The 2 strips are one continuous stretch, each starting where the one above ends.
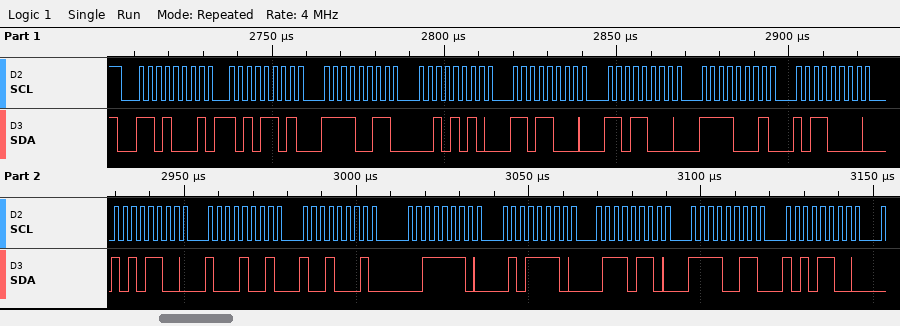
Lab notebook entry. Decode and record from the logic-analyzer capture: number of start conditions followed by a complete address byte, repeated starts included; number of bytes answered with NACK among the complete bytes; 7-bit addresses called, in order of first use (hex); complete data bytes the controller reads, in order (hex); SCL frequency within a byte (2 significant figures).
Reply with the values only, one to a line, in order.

1
0
0x68
AD F3 2A D8 D8 F1 B0 AC 89 91 3E 5E 76 F3 AC
400 kHz
